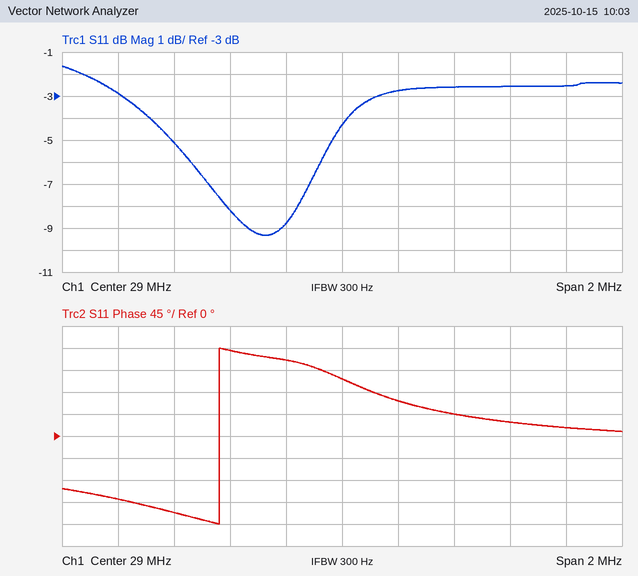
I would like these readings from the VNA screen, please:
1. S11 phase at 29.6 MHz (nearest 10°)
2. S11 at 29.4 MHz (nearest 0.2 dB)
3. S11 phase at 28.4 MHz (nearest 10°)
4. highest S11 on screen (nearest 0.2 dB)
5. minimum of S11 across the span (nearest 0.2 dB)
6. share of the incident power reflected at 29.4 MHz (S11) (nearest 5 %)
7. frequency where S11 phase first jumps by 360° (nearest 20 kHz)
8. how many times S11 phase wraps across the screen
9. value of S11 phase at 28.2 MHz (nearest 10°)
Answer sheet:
30°
-2.6 dB
-160°
-1.6 dB
-9.4 dB
55 %
28.56 MHz
1
-130°
